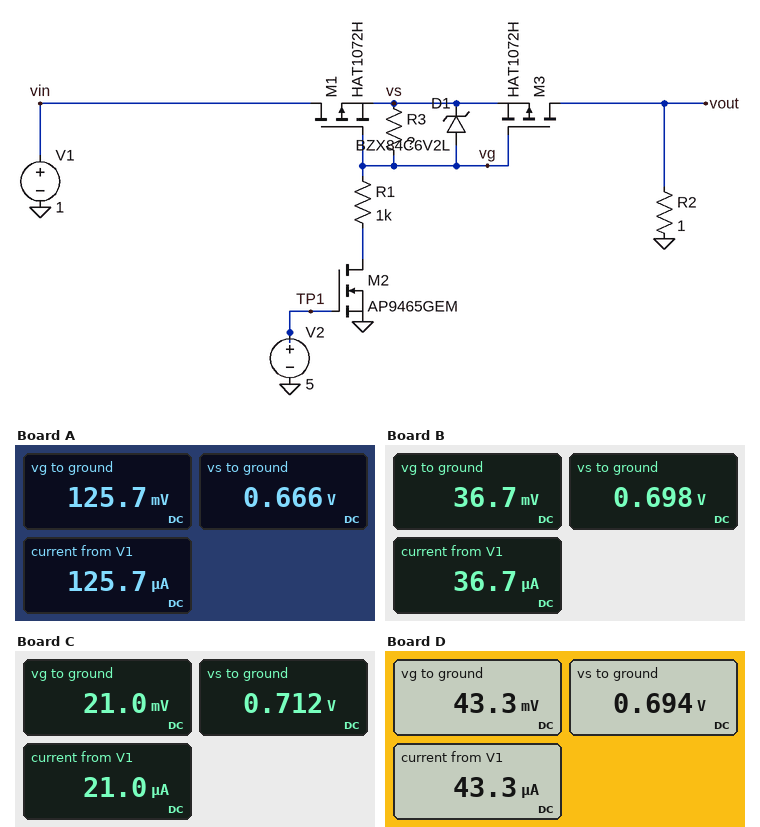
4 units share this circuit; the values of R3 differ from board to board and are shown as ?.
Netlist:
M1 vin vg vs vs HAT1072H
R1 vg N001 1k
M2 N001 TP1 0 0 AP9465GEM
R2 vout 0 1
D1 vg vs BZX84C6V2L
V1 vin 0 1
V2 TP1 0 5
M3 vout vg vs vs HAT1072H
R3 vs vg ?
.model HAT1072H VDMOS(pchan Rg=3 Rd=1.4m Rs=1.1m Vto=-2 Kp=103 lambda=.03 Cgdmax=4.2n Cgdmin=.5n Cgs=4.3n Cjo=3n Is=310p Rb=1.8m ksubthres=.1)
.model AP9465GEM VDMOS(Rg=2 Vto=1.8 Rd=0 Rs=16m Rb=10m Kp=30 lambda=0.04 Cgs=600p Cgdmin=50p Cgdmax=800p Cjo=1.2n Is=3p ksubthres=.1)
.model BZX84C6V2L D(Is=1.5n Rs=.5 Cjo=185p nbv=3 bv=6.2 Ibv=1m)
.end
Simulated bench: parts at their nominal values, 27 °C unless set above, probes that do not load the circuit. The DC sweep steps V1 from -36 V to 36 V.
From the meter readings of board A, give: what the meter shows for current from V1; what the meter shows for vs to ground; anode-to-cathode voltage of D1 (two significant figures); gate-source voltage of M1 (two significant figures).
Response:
125.7 µA
0.666 V
-540 mV
-540 mV
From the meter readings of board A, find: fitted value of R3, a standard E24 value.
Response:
4.3 kΩ
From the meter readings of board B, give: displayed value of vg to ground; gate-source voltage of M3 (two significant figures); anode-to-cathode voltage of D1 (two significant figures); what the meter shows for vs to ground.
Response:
36.7 mV
-660 mV
-660 mV
0.698 V
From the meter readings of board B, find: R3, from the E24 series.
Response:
18 kΩ
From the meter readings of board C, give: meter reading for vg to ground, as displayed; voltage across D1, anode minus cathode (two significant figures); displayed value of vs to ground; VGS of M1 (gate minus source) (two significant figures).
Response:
21.0 mV
-690 mV
0.712 V
-690 mV
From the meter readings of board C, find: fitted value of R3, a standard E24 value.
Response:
33 kΩ
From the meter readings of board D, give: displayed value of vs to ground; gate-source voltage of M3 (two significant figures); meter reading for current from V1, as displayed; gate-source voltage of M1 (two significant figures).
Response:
0.694 V
-650 mV
43.3 µA
-650 mV
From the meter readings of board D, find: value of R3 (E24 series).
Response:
15 kΩ
